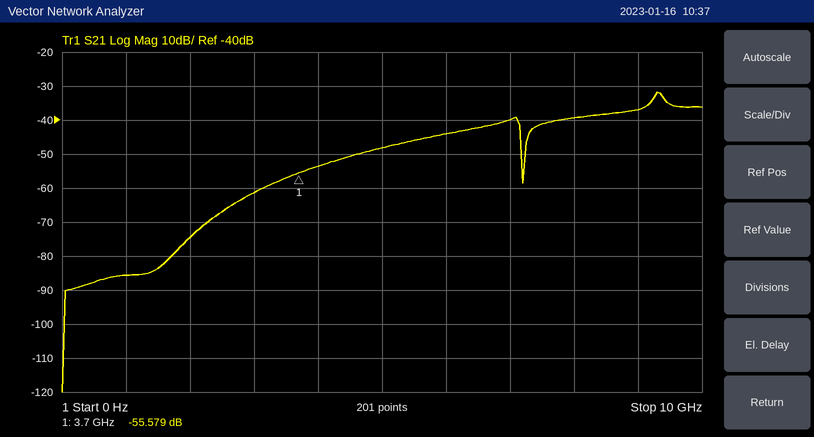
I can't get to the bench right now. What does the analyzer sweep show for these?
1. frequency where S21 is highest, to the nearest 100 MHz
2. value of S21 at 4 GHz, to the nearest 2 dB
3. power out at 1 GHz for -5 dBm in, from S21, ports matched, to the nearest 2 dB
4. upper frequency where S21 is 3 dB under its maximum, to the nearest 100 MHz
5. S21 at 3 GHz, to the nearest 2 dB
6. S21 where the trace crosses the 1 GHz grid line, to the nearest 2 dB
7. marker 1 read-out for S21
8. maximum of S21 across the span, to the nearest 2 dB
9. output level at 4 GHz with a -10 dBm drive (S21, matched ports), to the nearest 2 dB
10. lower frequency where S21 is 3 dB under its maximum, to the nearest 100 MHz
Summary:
9.3 GHz
-54 dB
-90 dBm
9.5 GHz
-62 dB
-86 dB
-55.579 dB
-32 dB
-64 dBm
9.2 GHz
